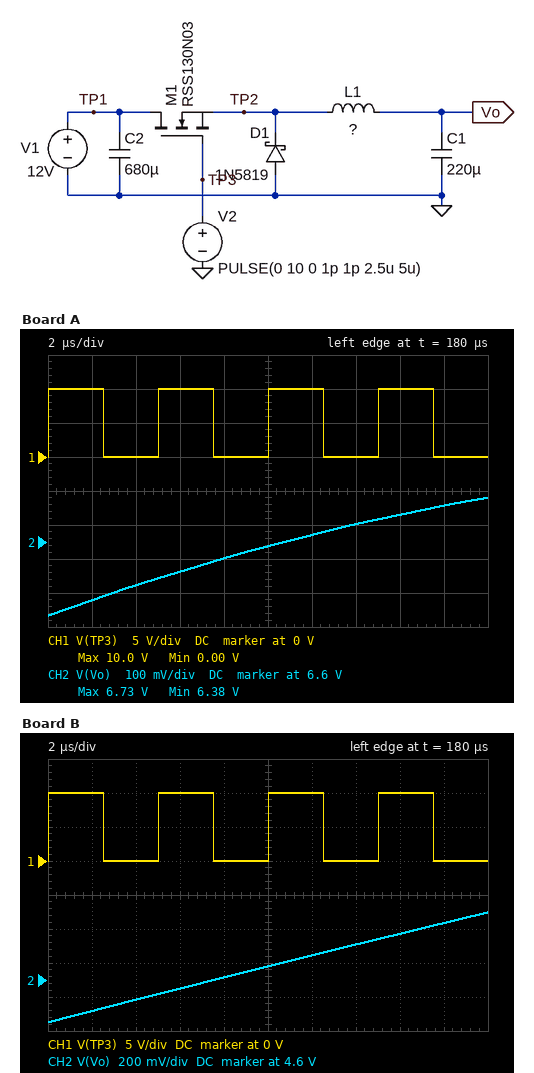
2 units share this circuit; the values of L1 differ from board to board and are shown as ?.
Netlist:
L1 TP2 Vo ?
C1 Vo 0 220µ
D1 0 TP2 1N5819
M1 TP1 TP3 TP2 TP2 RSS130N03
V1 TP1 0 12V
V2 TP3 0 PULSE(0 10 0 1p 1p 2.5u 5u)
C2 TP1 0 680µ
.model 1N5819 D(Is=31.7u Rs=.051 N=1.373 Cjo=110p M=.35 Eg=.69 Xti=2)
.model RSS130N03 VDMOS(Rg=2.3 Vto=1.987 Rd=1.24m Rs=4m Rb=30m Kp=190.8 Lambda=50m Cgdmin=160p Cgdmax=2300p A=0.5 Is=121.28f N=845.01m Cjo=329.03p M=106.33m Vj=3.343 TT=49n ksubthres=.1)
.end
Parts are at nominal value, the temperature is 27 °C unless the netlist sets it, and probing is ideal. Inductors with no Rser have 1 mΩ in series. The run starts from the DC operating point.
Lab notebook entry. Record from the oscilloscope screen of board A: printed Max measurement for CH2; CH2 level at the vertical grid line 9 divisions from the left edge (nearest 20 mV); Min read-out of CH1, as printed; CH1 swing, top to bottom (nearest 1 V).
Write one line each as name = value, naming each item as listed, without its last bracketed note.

printed Max measurement for CH2 = 6.73 V
CH2 level at the vertical grid line 9 divisions from the left edge = 6.70 V
Min read-out of CH1, as printed = 0.00 V
CH1 swing, top to bottom = 10 V
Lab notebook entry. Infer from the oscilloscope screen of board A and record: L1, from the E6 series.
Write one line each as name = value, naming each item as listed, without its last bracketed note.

L1, from the E6 series = 22 µH
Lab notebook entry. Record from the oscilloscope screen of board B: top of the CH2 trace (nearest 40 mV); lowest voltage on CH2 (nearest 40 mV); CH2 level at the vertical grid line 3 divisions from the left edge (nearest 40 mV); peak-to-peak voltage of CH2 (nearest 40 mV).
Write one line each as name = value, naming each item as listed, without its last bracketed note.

top of the CH2 trace = 5.00 V
lowest voltage on CH2 = 4.36 V
CH2 level at the vertical grid line 3 divisions from the left edge = 4.56 V
peak-to-peak voltage of CH2 = 640 mV
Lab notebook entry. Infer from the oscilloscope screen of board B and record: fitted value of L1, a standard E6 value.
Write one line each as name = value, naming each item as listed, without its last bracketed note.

fitted value of L1, a standard E6 value = 47 µH
